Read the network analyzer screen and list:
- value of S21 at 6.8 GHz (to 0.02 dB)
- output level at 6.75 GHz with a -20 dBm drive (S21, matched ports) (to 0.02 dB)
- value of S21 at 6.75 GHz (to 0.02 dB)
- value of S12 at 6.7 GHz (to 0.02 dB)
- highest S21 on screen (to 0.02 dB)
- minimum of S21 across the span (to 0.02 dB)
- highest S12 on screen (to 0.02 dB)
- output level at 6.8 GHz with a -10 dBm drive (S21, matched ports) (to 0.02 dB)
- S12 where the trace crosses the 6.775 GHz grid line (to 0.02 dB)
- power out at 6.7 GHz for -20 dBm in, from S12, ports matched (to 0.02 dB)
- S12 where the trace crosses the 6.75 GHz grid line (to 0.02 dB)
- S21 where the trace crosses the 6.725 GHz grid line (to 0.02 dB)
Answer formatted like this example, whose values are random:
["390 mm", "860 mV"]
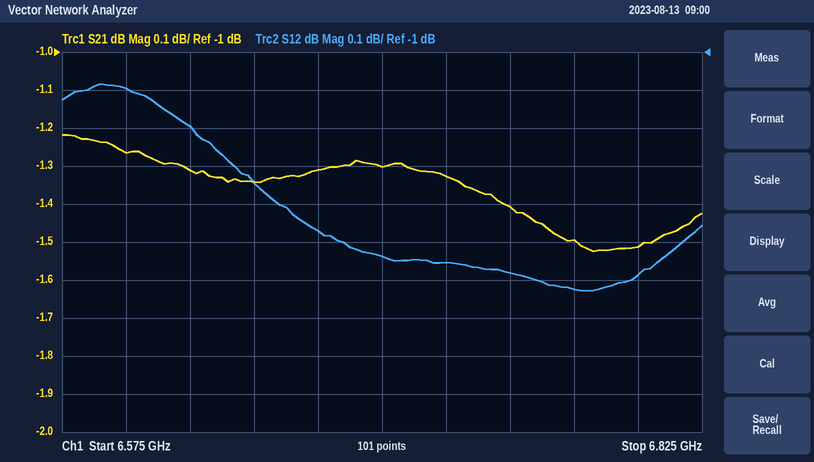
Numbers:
["-1.52 dB", "-21.40 dBm", "-1.40 dB", "-1.54 dB", "-1.22 dB", "-1.52 dB", "-1.08 dB", "-11.52 dBm", "-1.62 dB", "-21.54 dBm", "-1.58 dB", "-1.32 dB"]
